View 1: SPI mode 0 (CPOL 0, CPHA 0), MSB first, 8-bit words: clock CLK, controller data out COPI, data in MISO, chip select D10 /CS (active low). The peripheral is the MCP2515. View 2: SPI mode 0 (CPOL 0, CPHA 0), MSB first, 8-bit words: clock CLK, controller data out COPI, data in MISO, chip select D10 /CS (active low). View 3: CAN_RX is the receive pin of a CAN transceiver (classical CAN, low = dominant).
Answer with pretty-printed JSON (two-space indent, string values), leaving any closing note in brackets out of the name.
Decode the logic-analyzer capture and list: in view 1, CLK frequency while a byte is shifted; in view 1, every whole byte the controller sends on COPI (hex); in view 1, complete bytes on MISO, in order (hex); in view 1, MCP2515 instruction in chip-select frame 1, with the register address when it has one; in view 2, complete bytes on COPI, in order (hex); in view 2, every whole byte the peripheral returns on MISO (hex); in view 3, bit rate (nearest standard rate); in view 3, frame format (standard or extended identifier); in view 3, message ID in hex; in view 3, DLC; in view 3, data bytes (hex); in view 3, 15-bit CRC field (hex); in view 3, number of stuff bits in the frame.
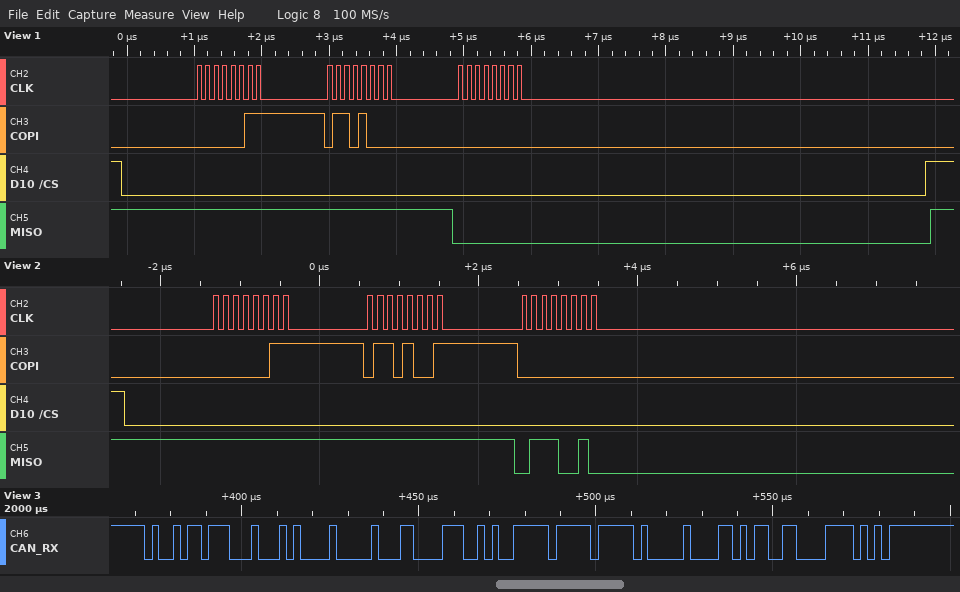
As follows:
{
  "in view 1, CLK frequency while a byte is shifted": "8 MHz",
  "in view 1, every whole byte the controller sends on COPI": "0x03 0x68 0x00",
  "in view 1, complete bytes on MISO, in order": "0xFF 0xFF 0x00",
  "in view 1, MCP2515 instruction in chip-select frame 1, with the register address when it has one": "READ 0x68",
  "in view 2, complete bytes on COPI, in order": "03 69 00",
  "in view 2, every whole byte the peripheral returns on MISO": "FF FF 72",
  "in view 3, bit rate": "500 kbit/s",
  "in view 3, frame format": "standard",
  "in view 3, message ID in hex": "0x4B7",
  "in view 3, DLC": "8",
  "in view 3, data bytes": "A1 00 C3 94 FF FF 00 6B",
  "in view 3, 15-bit CRC field": "0x187A",
  "in view 3, number of stuff bits in the frame": "5"
}
